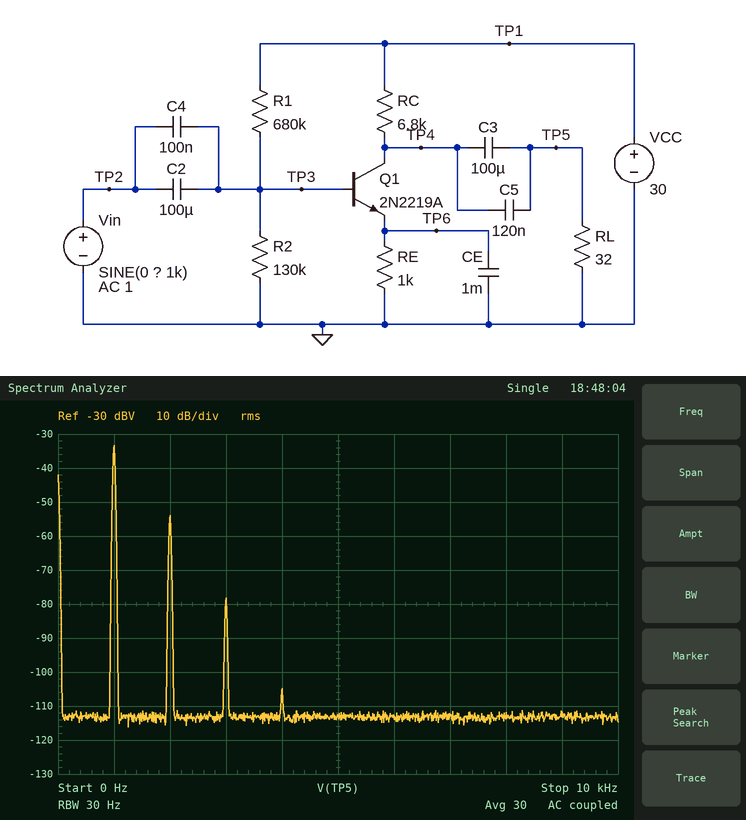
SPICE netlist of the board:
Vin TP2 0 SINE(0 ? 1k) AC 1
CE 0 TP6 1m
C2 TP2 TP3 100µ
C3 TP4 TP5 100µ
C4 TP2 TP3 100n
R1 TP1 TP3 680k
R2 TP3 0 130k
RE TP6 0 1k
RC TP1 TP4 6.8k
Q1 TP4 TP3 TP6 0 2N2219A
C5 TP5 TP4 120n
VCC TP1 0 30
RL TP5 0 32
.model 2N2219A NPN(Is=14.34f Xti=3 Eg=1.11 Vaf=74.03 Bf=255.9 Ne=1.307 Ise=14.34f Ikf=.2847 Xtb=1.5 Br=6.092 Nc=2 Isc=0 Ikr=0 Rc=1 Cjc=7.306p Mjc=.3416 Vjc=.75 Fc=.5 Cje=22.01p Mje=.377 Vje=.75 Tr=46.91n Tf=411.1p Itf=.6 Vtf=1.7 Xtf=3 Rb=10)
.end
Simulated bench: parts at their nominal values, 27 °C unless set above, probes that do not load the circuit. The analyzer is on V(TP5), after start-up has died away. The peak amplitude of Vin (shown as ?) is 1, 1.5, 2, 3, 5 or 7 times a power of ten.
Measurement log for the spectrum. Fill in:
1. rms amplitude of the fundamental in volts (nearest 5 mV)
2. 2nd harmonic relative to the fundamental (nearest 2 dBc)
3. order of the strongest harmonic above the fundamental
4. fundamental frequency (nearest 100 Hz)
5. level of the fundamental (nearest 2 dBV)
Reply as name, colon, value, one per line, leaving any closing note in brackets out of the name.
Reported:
rms amplitude of the fundamental in volts: 20 mV
2nd harmonic relative to the fundamental: -20 dBc
order of the strongest harmonic above the fundamental: 2
fundamental frequency: 1.0 kHz
level of the fundamental: -34 dBV
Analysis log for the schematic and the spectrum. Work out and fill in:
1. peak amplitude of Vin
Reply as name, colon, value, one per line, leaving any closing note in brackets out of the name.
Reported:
peak amplitude of Vin: 10 mV
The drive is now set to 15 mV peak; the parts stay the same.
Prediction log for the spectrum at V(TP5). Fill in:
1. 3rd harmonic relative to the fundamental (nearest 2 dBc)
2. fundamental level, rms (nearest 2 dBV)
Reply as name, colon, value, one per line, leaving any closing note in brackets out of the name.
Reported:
3rd harmonic relative to the fundamental: -38 dBc
fundamental level, rms: -30 dBV
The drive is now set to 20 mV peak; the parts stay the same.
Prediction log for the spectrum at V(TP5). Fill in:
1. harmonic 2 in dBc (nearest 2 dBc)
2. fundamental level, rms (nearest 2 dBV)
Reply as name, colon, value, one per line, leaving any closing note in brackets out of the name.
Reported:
harmonic 2 in dBc: -14 dBc
fundamental level, rms: -28 dBV
